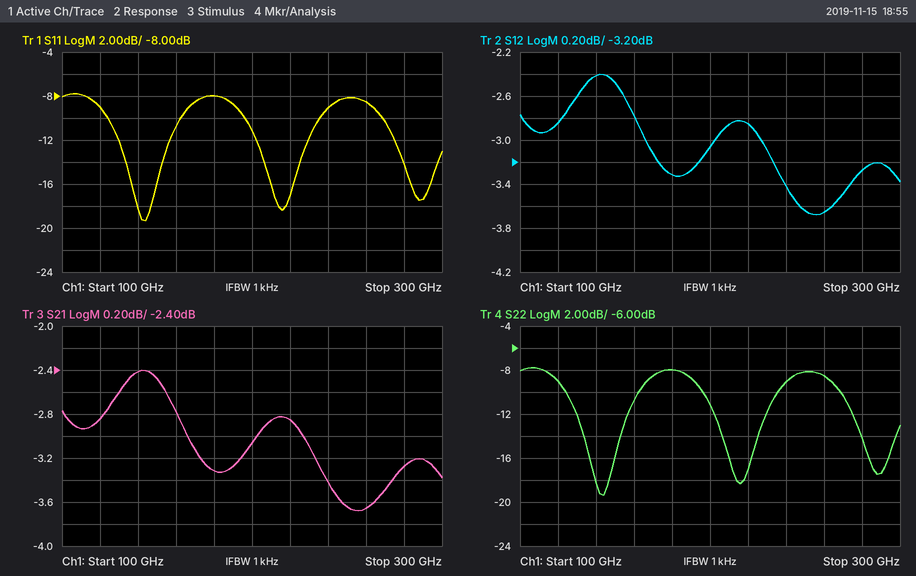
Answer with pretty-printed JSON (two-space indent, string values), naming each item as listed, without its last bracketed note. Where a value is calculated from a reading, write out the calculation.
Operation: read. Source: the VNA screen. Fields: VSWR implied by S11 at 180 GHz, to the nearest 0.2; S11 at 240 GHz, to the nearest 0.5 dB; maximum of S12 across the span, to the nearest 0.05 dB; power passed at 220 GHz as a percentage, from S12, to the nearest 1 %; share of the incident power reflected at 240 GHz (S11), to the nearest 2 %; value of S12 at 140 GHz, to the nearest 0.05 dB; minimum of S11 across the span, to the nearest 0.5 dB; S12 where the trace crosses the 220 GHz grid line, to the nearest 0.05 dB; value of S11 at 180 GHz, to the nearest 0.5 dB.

{
  "VSWR implied by S11 at 180 GHz, to the nearest 0.2": "|Γ| = 10^(-8/20) = 0.3981; VSWR = (1 + 0.3981)/(1 − 0.3981) ≈ 2.32, so 2.4 to the nearest 0.2",
  "S11 at 240 GHz, to the nearest 0.5 dB": "-9.0 dB",
  "maximum of S12 across the span, to the nearest 0.05 dB": "-2.40 dB",
  "power passed at 220 GHz as a percentage, from S12, to the nearest 1 %": "10^(-2.85/10) ≈ 52 %",
  "share of the incident power reflected at 240 GHz (S11), to the nearest 2 %": "10^(-9/10) ≈ 12.6 %, so 12 % to the nearest 2 %",
  "value of S12 at 140 GHz, to the nearest 0.05 dB": "-2.40 dB",
  "minimum of S11 across the span, to the nearest 0.5 dB": "-19.5 dB",
  "S12 where the trace crosses the 220 GHz grid line, to the nearest 0.05 dB": "-2.85 dB",
  "value of S11 at 180 GHz, to the nearest 0.5 dB": "-8.0 dB"
}
